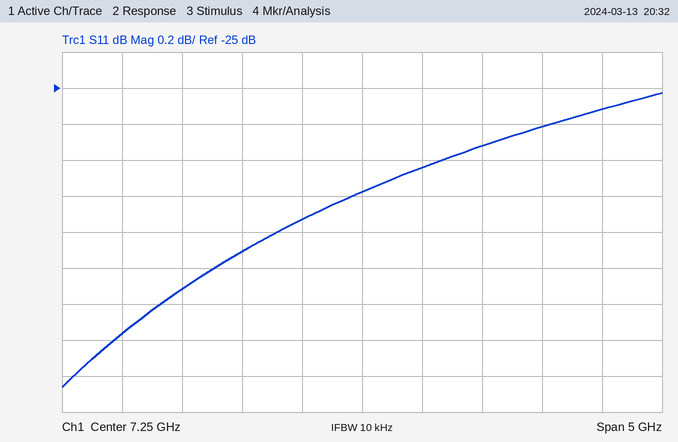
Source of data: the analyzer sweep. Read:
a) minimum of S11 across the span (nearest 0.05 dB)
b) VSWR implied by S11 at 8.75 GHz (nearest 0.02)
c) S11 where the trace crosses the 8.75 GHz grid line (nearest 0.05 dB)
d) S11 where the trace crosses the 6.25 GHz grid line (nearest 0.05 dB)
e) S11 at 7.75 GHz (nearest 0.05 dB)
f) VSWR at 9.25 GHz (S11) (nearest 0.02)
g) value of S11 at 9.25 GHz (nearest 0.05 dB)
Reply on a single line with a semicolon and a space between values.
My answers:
-26.65 dB; 1.12; -25.20 dB; -25.90 dB; -25.45 dB; 1.12; -25.10 dB
